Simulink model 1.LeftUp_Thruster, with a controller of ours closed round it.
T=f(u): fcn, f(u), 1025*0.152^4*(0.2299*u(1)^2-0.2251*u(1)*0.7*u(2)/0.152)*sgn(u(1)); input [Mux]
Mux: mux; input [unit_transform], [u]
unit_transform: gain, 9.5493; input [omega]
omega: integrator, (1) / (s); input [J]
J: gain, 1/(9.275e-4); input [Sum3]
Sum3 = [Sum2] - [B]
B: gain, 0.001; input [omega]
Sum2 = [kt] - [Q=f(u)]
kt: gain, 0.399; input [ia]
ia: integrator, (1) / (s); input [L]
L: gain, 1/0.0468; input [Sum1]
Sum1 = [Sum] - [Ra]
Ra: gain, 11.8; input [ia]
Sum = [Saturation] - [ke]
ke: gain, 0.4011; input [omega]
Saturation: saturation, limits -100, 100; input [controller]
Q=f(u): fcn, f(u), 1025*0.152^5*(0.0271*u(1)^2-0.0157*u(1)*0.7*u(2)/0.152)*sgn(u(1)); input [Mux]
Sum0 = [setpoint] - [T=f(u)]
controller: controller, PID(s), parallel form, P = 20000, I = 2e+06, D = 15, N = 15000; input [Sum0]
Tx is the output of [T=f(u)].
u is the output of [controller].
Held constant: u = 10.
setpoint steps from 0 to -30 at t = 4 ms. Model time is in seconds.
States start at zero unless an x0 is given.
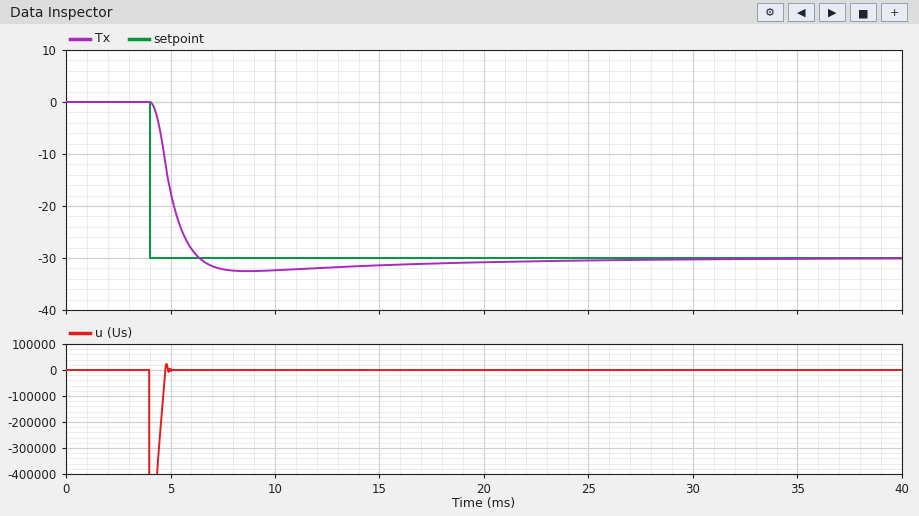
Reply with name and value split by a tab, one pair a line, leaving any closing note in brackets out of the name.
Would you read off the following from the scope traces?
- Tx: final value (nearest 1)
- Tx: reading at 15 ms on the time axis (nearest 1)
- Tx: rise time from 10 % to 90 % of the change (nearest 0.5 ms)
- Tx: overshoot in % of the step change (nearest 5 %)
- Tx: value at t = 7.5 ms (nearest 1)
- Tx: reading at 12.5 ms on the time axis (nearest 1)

Tx: final value	-30
Tx: reading at 15 ms on the time axis	-31
Tx: rise time from 10 % to 90 % of the change	1.5 ms
Tx: overshoot in % of the step change	10 %
Tx: value at t = 7.5 ms	-32
Tx: reading at 12.5 ms on the time axis	-32
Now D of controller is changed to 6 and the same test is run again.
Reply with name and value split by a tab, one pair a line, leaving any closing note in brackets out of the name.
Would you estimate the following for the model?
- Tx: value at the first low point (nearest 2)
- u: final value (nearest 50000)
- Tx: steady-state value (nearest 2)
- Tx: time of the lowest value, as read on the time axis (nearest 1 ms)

Tx: value at the first low point	-32
u: final value	0
Tx: steady-state value	-30
Tx: time of the lowest value, as read on the time axis	7 ms
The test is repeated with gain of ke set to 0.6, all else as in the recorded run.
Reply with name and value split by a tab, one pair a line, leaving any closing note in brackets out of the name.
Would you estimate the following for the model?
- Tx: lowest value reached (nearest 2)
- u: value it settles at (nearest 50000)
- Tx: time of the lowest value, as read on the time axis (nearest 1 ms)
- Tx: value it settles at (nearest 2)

Tx: lowest value reached	-32
u: value it settles at	0
Tx: time of the lowest value, as read on the time axis	9 ms
Tx: value it settles at	-30
